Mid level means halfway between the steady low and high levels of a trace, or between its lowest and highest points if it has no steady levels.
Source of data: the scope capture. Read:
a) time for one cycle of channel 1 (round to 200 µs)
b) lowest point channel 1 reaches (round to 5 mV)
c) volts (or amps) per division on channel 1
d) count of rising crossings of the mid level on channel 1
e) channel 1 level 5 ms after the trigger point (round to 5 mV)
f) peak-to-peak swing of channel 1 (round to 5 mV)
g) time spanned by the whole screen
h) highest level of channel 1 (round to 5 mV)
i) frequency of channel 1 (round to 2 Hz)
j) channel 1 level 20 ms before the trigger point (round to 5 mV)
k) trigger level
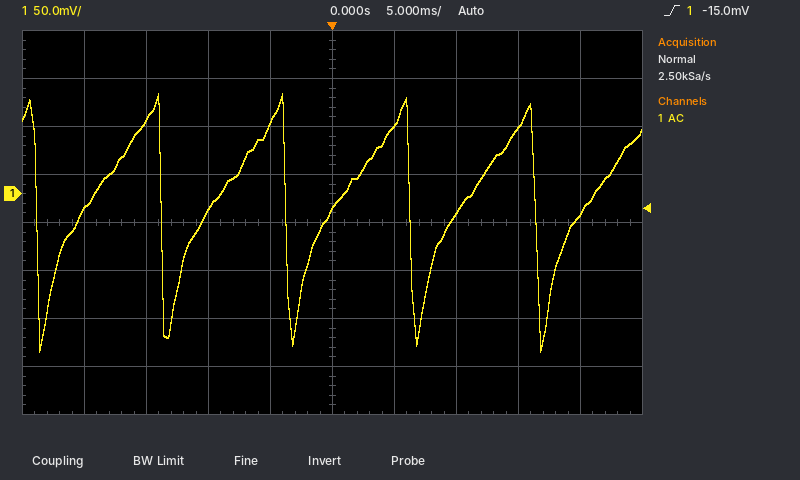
10.0 ms
-165 mV
50 mV
5
70 mV
270 mV
50 ms
105 mV
100 Hz
-15 mV
-15.0 mV
